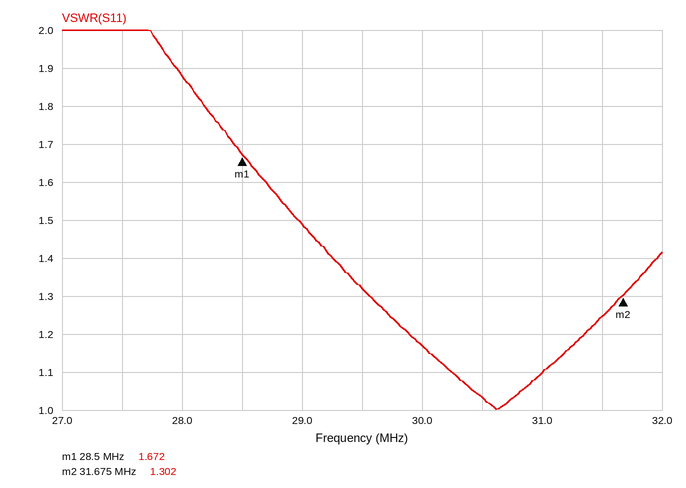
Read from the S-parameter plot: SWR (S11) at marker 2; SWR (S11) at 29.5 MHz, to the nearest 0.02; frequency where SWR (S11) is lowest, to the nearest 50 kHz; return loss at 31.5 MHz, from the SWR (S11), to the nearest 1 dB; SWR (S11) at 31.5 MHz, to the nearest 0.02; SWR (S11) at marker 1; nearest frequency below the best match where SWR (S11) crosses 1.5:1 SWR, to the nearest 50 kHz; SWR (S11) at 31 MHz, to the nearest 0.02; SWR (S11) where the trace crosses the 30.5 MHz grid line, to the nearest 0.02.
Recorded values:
1.302
1.32
30.60 MHz
19 dB
1.24
1.672
28.95 MHz
1.10
1.04
